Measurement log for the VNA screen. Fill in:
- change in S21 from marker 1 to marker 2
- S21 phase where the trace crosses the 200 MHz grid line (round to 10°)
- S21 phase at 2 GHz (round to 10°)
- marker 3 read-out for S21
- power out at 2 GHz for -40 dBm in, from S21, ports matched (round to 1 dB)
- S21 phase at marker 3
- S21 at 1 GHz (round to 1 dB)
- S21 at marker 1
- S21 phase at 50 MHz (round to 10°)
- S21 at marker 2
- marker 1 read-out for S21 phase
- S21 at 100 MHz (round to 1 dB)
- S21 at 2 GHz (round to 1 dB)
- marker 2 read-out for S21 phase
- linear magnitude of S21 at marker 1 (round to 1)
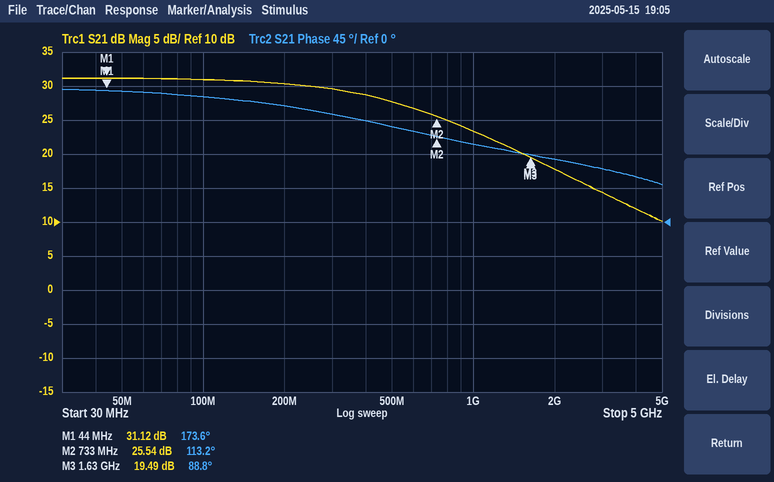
-5.58 dB
150°
80°
19.49 dB
-22 dBm
88.8°
23 dB
31.12 dB
170°
25.54 dB
173.6°
31 dB
18 dB
113.2°
36
